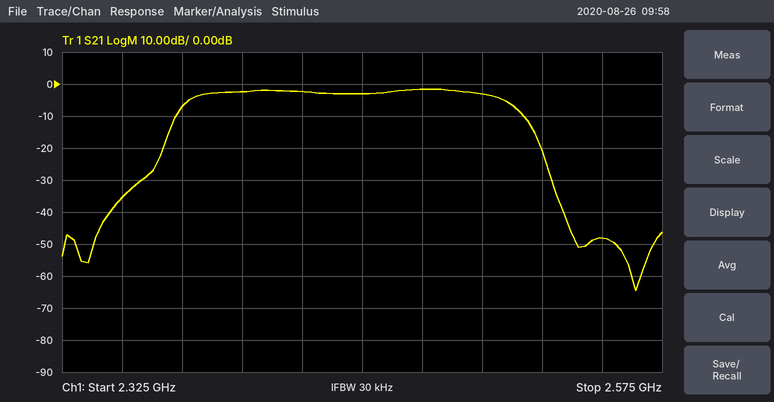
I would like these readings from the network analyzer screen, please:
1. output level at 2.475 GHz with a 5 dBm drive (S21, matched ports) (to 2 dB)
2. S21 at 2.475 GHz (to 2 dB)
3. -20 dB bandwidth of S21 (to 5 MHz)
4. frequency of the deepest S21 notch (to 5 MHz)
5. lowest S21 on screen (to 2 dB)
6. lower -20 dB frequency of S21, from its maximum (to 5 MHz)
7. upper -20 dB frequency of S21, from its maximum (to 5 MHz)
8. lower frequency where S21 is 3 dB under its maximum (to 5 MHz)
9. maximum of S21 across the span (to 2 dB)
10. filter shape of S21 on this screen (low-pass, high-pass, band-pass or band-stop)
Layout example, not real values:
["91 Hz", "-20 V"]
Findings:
["4 dBm", "-2 dB", "160 MHz", "2.565 GHz", "-64 dB", "2.365 GHz", "2.525 GHz", "2.380 GHz", "-2 dB", "band-pass"]
